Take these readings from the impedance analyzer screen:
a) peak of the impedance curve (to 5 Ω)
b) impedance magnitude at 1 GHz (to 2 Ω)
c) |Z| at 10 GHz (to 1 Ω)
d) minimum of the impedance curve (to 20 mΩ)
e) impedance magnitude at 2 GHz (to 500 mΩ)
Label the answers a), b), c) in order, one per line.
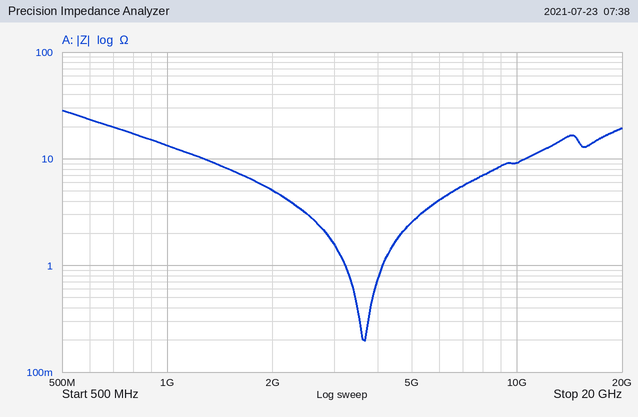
a) 30 Ω
b) 14 Ω
c) 9 Ω
d) 200 mΩ
e) 5.0 Ω
